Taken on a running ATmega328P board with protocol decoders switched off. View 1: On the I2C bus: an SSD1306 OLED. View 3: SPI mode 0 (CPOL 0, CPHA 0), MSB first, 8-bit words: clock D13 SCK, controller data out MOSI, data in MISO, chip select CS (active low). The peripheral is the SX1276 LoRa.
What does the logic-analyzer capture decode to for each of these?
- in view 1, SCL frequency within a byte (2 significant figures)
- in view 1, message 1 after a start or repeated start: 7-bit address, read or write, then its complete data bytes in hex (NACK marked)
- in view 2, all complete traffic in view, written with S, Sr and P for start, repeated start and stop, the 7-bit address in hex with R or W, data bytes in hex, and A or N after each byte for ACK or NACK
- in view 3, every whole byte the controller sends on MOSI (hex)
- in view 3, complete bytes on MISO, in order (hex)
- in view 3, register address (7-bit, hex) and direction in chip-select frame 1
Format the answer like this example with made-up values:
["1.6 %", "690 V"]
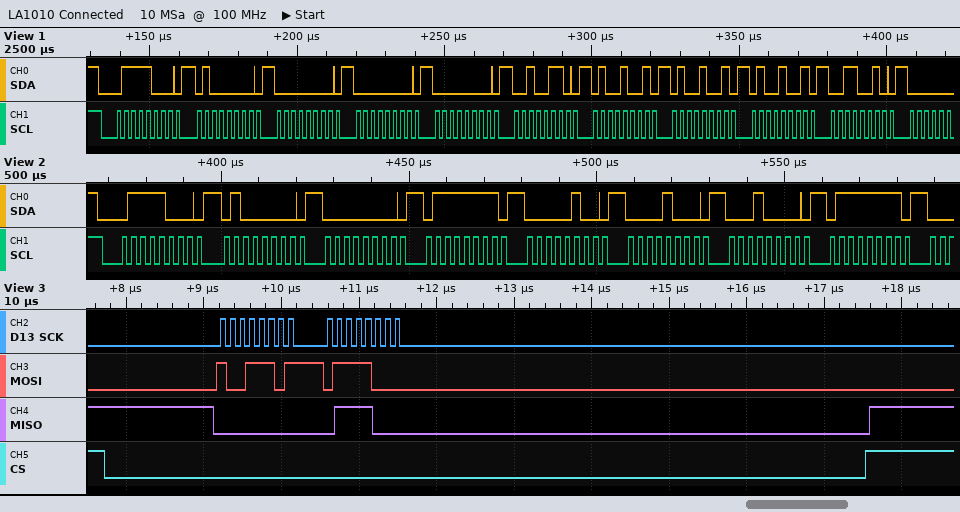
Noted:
["400 kHz", "0x3C write: 40 00 00 00 26 49 49 49 32", "S 3CW A 40 A 00 A 7F A 04 A 08 A 10 A 7F A", "9D 78", "00 78", "0x1D write"]
